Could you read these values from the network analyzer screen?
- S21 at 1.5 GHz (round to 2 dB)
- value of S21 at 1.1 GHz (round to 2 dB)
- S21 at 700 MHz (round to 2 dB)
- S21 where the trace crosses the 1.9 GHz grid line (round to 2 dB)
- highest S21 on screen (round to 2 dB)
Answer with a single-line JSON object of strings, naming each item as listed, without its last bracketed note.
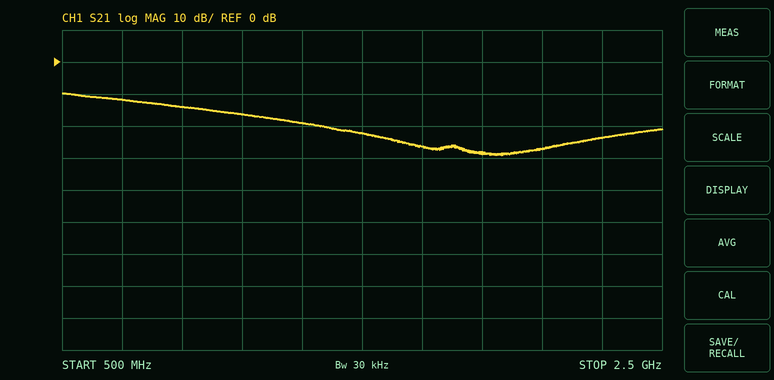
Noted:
{"S21 at 1.5 GHz": "-22 dB", "value of S21 at 1.1 GHz": "-16 dB", "S21 at 700 MHz": "-12 dB", "S21 where the trace crosses the 1.9 GHz grid line": "-28 dB", "highest S21 on screen": "-10 dB"}
